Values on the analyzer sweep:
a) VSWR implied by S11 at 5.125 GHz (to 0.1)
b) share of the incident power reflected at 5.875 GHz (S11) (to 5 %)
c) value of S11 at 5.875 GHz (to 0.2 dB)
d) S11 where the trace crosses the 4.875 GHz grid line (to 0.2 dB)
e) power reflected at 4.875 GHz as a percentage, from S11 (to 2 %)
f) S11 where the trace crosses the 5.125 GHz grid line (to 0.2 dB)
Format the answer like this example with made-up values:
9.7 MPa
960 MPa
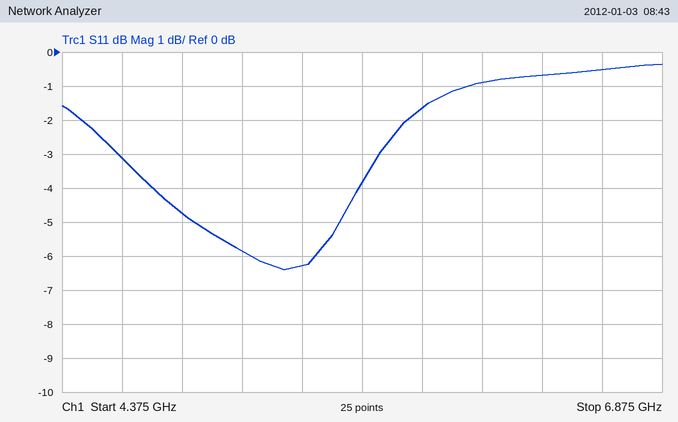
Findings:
3.1
70 %
-1.6 dB
-4.8 dB
34 %
-5.8 dB
